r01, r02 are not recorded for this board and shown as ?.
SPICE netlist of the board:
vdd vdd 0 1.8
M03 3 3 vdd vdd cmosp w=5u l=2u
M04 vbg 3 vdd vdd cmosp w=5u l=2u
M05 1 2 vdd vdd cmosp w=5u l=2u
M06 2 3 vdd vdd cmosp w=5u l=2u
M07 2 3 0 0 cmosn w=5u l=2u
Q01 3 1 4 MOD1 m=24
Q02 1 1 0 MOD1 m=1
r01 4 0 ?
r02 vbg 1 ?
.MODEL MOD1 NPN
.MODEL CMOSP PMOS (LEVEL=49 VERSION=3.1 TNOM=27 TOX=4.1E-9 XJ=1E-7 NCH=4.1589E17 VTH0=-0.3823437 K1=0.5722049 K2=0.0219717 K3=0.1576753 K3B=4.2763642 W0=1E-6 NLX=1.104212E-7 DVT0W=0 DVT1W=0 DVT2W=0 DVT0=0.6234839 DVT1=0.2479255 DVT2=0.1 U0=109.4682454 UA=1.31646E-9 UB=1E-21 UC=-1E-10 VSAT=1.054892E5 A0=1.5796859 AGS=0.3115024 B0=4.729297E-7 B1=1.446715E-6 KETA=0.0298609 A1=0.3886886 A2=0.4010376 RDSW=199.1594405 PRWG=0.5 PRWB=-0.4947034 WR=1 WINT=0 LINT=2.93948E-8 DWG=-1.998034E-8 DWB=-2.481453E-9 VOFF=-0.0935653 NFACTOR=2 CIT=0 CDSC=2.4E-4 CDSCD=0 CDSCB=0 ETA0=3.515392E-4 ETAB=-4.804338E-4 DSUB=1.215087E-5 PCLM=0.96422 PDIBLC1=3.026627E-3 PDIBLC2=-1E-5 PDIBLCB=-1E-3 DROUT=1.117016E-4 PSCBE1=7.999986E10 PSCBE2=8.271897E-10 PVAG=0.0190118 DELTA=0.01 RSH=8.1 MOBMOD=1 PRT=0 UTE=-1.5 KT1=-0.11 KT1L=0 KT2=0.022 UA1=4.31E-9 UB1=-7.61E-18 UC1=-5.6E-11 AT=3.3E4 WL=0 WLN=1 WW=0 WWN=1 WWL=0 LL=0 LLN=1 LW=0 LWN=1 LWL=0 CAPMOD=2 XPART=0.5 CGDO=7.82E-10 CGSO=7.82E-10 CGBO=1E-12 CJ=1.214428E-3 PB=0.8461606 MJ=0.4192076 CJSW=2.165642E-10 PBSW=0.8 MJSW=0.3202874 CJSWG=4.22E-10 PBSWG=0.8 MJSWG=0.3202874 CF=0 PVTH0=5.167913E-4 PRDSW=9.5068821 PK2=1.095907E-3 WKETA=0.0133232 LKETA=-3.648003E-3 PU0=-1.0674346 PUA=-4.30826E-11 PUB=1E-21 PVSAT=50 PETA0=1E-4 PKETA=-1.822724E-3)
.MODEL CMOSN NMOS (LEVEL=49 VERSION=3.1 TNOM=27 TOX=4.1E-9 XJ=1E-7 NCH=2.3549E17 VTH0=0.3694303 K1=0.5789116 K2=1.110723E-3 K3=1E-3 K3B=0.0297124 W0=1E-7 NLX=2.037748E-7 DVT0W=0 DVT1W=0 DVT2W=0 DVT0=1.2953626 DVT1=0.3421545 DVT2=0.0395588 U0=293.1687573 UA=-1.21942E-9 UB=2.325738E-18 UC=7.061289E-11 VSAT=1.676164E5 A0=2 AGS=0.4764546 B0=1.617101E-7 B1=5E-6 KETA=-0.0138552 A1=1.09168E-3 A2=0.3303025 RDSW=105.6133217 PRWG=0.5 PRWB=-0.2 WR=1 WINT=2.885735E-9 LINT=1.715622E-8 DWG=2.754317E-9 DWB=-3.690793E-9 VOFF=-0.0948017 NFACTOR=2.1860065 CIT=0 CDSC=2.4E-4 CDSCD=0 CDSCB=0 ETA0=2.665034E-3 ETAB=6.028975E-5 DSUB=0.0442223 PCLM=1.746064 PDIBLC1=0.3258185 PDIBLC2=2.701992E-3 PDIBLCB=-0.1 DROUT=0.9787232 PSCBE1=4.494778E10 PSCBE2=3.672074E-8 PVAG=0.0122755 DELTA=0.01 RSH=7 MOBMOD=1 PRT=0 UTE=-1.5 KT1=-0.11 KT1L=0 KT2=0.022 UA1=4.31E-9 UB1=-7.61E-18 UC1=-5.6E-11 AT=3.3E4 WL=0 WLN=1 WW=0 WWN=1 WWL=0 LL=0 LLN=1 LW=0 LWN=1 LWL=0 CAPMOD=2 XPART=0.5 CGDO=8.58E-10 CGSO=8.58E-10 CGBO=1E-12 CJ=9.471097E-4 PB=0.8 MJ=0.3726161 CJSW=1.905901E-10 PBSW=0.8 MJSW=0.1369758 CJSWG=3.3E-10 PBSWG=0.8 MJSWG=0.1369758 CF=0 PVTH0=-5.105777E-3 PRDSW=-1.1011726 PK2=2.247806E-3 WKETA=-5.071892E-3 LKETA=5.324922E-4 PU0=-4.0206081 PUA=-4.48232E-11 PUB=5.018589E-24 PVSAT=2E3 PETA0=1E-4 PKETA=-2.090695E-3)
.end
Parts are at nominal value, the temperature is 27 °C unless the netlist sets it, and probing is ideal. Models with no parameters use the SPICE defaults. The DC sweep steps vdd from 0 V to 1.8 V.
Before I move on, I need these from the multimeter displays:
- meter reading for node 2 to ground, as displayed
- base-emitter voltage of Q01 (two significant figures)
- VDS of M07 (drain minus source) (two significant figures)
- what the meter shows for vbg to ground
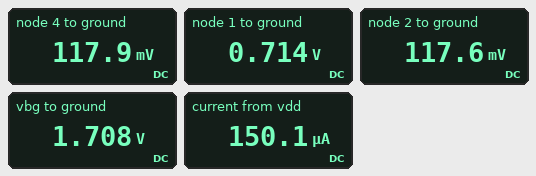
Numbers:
117.6 mV
600 mV
120 mV
1.708 V
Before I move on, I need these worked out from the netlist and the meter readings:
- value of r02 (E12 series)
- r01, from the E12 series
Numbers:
120 kΩ
4.7 kΩ
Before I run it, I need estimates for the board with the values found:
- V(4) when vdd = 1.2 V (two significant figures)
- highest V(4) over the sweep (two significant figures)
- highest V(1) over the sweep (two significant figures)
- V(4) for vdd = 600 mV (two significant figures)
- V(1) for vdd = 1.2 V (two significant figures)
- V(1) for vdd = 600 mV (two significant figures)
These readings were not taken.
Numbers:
55 mV
120 mV
710 mV
8.2 mV
630 mV
540 mV
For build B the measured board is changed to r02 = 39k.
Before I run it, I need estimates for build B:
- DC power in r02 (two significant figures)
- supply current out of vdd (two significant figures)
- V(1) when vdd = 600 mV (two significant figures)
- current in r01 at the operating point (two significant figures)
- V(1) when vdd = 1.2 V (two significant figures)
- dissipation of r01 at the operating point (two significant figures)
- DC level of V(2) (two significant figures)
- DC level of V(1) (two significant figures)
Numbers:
16 µW
160 µA
550 mV
26 µA
650 mV
3.1 µW
120 mV
720 mV
